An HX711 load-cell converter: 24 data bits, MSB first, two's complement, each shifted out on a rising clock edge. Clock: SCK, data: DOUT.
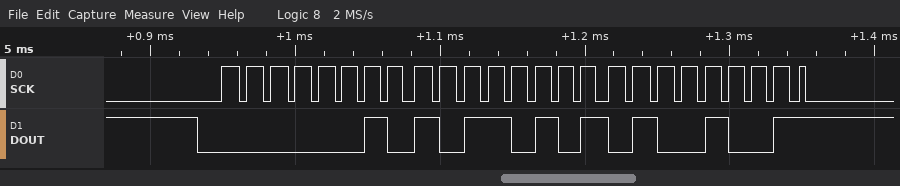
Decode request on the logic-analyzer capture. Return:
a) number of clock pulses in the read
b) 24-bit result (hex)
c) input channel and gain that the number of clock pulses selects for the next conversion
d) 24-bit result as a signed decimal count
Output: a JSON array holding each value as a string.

["25", "0x02B549", "channel A, gain 128", "177481"]
